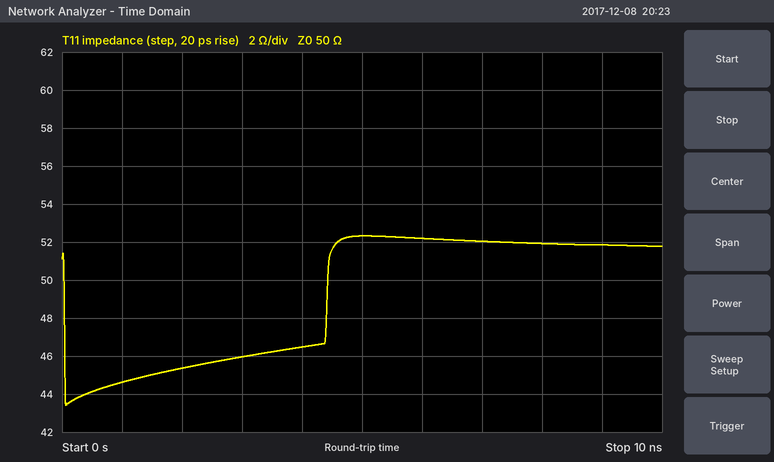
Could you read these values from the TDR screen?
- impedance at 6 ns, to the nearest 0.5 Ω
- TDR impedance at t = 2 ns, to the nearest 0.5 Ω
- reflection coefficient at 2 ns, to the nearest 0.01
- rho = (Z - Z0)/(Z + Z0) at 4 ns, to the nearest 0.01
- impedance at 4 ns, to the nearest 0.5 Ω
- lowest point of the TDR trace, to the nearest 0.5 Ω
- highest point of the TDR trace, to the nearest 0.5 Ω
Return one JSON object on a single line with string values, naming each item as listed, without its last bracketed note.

{"impedance at 6 ns, to the nearest 0.5 Ω": "52.0 Ω", "TDR impedance at t = 2 ns, to the nearest 0.5 Ω": "45.5 Ω", "reflection coefficient at 2 ns, to the nearest 0.01": "-0.05", "rho = (Z - Z0)/(Z + Z0) at 4 ns, to the nearest 0.01": "-0.04", "impedance at 4 ns, to the nearest 0.5 Ω": "46.5 Ω", "lowest point of the TDR trace, to the nearest 0.5 Ω": "43.5 Ω", "highest point of the TDR trace, to the nearest 0.5 Ω": "52.5 Ω"}
